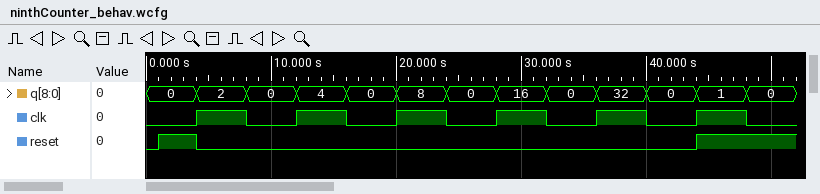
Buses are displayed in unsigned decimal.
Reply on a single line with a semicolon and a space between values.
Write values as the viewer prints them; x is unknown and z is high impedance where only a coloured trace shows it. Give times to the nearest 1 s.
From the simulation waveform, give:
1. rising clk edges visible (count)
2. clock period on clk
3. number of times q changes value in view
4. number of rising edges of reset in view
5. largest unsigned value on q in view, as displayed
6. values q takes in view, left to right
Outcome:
6; 8 s; 12; 2; 32; 0, 2, 0, 4, 0, 8, 0, 16, 0, 32, 0, 1, 0
